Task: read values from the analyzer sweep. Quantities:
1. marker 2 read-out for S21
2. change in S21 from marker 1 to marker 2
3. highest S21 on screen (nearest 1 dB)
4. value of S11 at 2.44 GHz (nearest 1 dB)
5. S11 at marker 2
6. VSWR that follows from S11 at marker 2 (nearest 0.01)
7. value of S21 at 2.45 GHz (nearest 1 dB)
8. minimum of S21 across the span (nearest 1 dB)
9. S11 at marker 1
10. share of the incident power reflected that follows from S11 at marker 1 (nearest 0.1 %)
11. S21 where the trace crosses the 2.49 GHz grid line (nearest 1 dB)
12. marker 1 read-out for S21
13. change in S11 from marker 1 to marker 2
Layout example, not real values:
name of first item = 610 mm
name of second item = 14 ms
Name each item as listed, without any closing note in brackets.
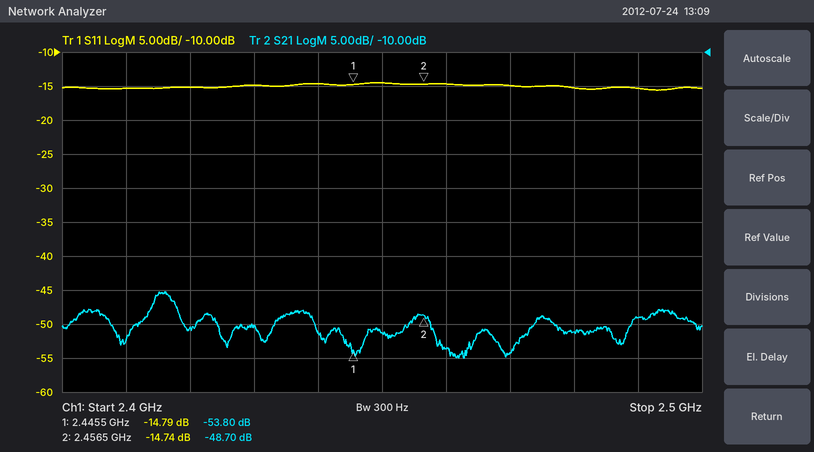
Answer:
marker 2 read-out for S21 = -48.70 dB
change in S21 from marker 1 to marker 2 = 5.10 dB
highest S21 on screen = -45 dB
value of S11 at 2.44 GHz = -15 dB
S11 at marker 2 = -14.74 dB
VSWR that follows from S11 at marker 2 = 1.45
value of S21 at 2.45 GHz = -51 dB
minimum of S21 across the span = -55 dB
S11 at marker 1 = -14.79 dB
share of the incident power reflected that follows from S11 at marker 1 = 3.3 %
S21 where the trace crosses the 2.49 GHz grid line = -49 dB
marker 1 read-out for S21 = -53.80 dB
change in S11 from marker 1 to marker 2 = 0.05 dB
